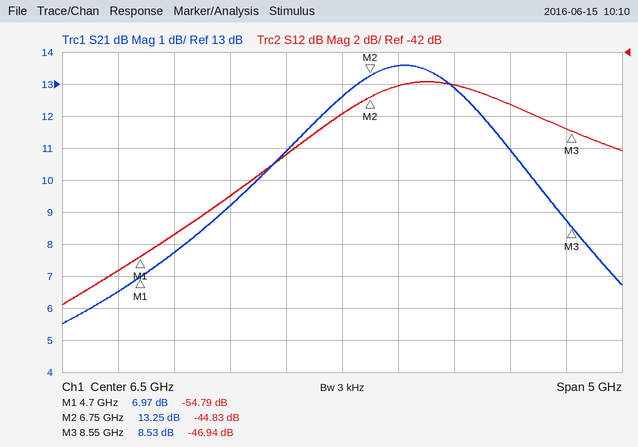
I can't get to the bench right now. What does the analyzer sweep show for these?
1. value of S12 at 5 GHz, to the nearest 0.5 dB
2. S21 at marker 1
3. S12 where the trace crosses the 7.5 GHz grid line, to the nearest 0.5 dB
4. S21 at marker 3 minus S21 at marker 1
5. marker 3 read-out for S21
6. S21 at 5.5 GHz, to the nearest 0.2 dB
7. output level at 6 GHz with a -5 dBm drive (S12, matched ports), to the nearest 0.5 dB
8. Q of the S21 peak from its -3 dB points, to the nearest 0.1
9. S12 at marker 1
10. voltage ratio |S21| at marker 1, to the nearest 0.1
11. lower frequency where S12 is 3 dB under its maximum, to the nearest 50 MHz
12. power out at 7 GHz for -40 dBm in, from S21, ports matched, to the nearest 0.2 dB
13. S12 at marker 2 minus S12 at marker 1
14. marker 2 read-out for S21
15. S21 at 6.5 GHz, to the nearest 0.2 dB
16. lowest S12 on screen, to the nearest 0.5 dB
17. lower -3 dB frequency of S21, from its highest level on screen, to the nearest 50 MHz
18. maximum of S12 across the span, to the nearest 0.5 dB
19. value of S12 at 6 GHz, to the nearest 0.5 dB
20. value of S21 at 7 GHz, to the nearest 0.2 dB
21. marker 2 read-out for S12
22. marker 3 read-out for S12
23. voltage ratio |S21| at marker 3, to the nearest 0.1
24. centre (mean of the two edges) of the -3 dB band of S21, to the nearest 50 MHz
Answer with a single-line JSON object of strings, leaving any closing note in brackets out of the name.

{"value of S12 at 5 GHz, to the nearest 0.5 dB": "-53.5 dB", "S21 at marker 1": "6.97 dB", "S12 where the trace crosses the 7.5 GHz grid line, to the nearest 0.5 dB": "-44.0 dB", "S21 at marker 3 minus S21 at marker 1": "1.56 dB", "marker 3 read-out for S21": "8.53 dB", "S21 at 5.5 GHz, to the nearest 0.2 dB": "9.2 dB", "output level at 6 GHz with a -5 dBm drive (S12, matched ports), to the nearest 0.5 dB": "-53.5 dBm", "Q of the S21 peak from its -3 dB points, to the nearest 0.1": "3.2", "S12 at marker 1": "-54.79 dB", "voltage ratio |S21| at marker 1, to the nearest 0.1": "2.2", "lower frequency where S12 is 3 dB under its maximum, to the nearest 50 MHz": "6.30 GHz", "power out at 7 GHz for -40 dBm in, from S21, ports matched, to the nearest 0.2 dB": "-26.4 dBm", "S12 at marker 2 minus S12 at marker 1": "9.96 dB", "marker 2 read-out for S21": "13.25 dB", "S21 at 6.5 GHz, to the nearest 0.2 dB": "12.6 dB", "lowest S12 on screen, to the nearest 0.5 dB": "-58.0 dB", "lower -3 dB frequency of S21, from its highest level on screen, to the nearest 50 MHz": "5.90 GHz", "maximum of S12 across the span, to the nearest 0.5 dB": "-44.0 dB", "value of S12 at 6 GHz, to the nearest 0.5 dB": "-48.5 dB", "value of S21 at 7 GHz, to the nearest 0.2 dB": "13.6 dB", "marker 2 read-out for S12": "-44.83 dB", "marker 3 read-out for S12": "-46.94 dB", "voltage ratio |S21| at marker 3, to the nearest 0.1": "2.7", "centre (mean of the two edges) of the -3 dB band of S21, to the nearest 50 MHz": "7.00 GHz"}
